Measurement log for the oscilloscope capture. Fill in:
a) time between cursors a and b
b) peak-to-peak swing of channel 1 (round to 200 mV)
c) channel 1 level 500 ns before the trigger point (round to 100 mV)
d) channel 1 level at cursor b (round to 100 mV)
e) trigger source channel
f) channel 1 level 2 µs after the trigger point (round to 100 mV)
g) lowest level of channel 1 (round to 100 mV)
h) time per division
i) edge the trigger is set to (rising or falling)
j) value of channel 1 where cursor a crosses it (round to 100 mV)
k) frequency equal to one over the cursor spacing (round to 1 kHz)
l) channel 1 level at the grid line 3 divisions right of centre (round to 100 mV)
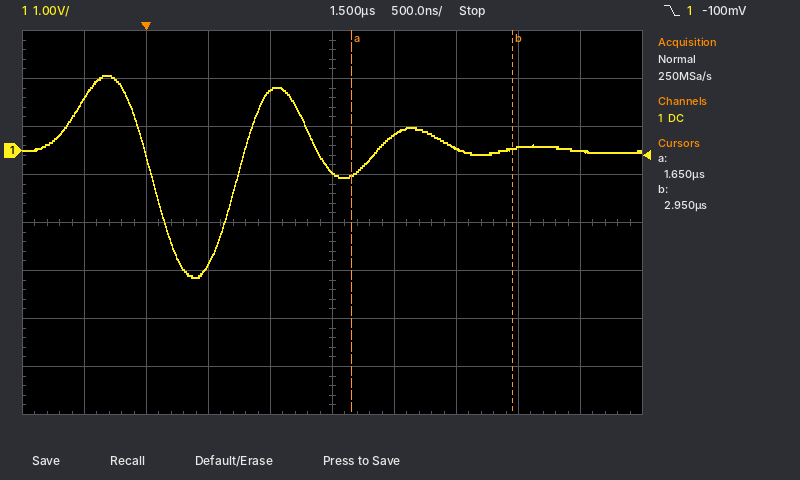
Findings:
1.30 µs
4.2 V
1.1 V
0.0 V
channel 1
300 mV
-2.6 V
500 ns
falling
-500 mV
769 kHz
100 mV
